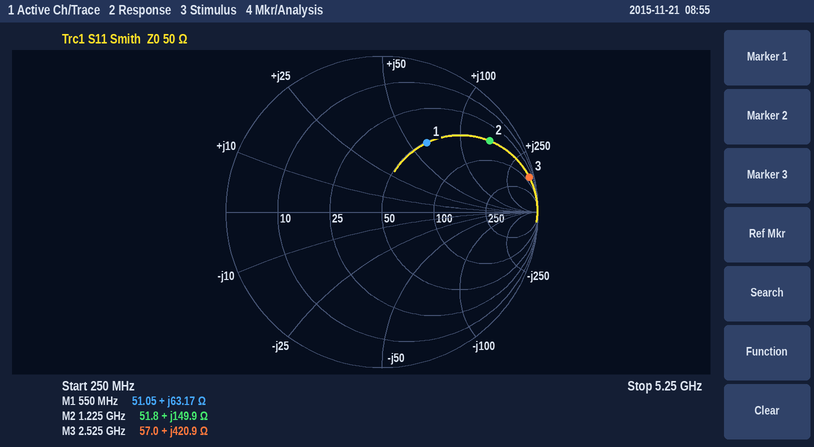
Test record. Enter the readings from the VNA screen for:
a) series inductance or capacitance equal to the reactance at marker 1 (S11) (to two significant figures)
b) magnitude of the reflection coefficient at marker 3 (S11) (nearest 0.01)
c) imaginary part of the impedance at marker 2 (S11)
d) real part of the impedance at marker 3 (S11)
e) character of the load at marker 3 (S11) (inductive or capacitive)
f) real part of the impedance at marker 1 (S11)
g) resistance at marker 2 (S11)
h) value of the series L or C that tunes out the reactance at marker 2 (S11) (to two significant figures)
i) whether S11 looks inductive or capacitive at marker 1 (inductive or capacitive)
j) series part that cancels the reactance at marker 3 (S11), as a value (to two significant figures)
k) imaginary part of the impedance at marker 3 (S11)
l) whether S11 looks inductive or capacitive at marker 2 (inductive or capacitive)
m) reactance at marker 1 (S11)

18 nH
0.97
+149.9 Ω
57.0 Ω
inductive
51.05 Ω
51.8 Ω
870 fF
inductive
150 fF
+420.9 Ω
inductive
+63.17 Ω
